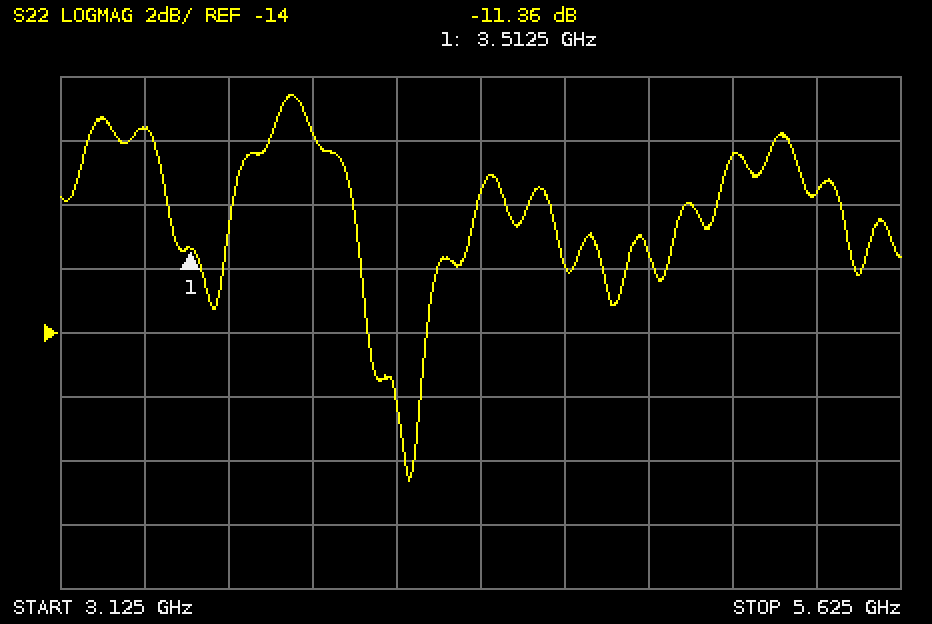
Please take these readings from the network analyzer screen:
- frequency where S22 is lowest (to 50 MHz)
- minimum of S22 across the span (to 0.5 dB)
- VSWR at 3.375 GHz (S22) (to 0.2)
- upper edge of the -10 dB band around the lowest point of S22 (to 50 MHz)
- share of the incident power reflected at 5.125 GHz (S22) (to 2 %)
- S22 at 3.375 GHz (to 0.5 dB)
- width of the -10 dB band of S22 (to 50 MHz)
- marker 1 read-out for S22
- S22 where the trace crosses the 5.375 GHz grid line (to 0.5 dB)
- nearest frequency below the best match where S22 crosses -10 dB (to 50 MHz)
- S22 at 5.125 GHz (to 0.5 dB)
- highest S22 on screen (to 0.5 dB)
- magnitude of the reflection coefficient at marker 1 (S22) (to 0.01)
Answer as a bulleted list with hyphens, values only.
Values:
- 4.15 GHz
- -18.5 dB
- 2.4
- 4.35 GHz
- 14 %
- -7.5 dB
- 350 MHz
- -11.36 dB
- -9.5 dB
- 4.00 GHz
- -8.5 dB
- -6.5 dB
- 0.27
